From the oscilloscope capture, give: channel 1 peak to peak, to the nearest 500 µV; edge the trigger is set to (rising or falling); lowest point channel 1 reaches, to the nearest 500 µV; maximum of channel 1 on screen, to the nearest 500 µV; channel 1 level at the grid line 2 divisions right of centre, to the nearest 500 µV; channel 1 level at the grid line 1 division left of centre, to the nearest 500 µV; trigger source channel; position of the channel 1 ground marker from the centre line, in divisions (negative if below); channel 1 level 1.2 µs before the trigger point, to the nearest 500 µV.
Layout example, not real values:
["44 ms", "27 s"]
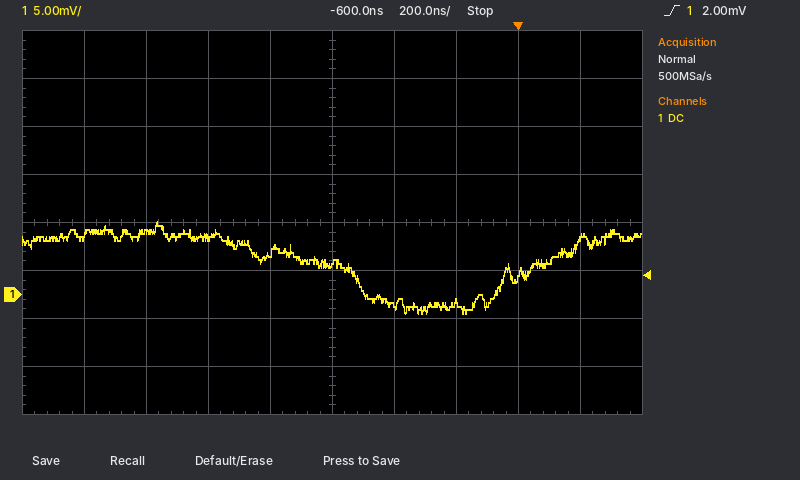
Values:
["9.5 mV", "rising", "-2.0 mV", "7.5 mV", "-1.0 mV", "4.5 mV", "channel 1", "-1.5 div", "6.5 mV"]
